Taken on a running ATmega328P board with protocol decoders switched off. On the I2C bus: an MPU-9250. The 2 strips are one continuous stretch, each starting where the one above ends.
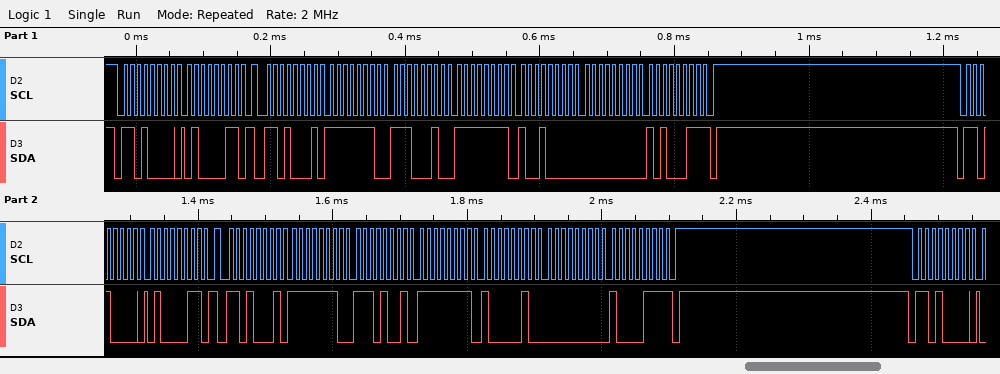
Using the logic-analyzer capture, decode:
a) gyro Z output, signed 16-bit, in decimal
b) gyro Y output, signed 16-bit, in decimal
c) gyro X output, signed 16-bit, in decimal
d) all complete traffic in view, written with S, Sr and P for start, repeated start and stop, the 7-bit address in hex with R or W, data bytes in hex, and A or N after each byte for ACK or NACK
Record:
163
-112
-286
S 68W A 43 A Sr 68R A FE A E2 A FF A 90 A 00 A A3 N P S 68W A 43 A Sr 68R A FE A E9 A FF A 82 A 00 A 87 N P S 68W A
